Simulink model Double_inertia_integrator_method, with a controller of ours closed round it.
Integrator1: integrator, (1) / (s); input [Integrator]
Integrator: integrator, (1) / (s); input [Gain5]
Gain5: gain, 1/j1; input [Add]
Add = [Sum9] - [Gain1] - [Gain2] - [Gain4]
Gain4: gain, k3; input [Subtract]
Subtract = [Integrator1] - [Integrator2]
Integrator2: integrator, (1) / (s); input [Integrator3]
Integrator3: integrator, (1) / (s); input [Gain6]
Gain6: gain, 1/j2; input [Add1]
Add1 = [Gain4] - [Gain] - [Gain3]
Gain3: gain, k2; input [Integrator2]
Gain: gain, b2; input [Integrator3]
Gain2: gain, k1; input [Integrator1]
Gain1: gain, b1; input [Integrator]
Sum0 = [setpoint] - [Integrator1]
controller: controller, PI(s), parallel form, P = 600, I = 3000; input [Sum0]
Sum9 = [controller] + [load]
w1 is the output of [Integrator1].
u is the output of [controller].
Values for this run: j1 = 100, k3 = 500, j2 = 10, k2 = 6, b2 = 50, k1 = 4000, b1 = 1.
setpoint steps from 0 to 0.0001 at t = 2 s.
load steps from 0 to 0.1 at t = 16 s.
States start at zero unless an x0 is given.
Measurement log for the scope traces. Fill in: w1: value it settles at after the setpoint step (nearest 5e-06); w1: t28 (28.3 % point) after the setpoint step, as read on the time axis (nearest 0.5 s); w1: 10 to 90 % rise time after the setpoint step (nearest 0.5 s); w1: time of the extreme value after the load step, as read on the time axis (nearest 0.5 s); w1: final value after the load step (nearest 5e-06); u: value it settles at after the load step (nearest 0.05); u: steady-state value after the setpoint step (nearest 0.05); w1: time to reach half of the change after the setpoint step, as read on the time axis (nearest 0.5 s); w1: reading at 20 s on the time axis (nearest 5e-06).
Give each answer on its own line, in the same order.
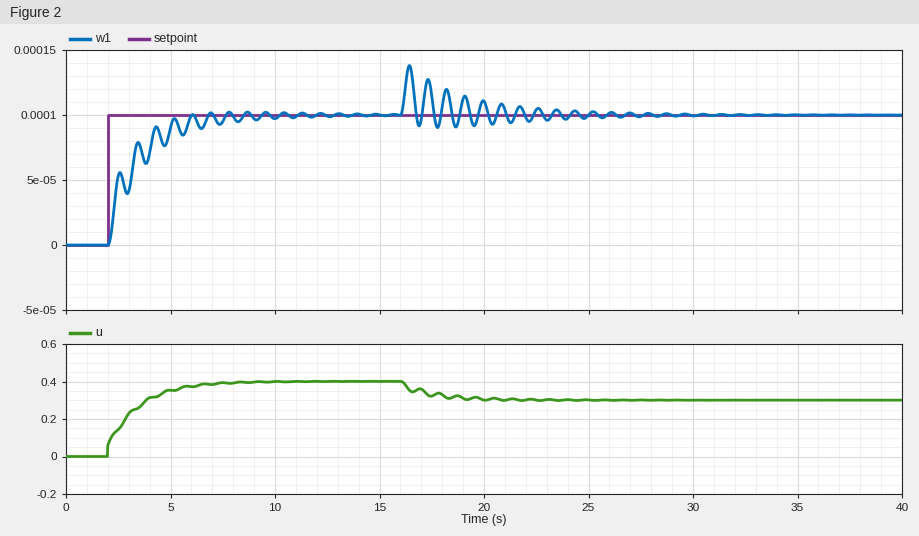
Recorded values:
0.000100
2.5 s
2.0 s
16.5 s
0.000100
0.30
0.40
2.5 s
0.000110
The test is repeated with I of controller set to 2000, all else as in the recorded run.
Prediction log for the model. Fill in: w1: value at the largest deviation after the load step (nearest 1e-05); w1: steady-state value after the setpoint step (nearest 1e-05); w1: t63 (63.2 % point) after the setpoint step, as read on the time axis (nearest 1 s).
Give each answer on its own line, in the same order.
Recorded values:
0.00014
0.00010
4 s
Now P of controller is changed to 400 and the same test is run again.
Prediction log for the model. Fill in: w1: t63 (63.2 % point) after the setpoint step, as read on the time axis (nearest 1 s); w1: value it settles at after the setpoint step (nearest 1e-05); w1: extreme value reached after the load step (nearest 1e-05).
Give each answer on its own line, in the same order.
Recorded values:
3 s
0.00010
0.00014
